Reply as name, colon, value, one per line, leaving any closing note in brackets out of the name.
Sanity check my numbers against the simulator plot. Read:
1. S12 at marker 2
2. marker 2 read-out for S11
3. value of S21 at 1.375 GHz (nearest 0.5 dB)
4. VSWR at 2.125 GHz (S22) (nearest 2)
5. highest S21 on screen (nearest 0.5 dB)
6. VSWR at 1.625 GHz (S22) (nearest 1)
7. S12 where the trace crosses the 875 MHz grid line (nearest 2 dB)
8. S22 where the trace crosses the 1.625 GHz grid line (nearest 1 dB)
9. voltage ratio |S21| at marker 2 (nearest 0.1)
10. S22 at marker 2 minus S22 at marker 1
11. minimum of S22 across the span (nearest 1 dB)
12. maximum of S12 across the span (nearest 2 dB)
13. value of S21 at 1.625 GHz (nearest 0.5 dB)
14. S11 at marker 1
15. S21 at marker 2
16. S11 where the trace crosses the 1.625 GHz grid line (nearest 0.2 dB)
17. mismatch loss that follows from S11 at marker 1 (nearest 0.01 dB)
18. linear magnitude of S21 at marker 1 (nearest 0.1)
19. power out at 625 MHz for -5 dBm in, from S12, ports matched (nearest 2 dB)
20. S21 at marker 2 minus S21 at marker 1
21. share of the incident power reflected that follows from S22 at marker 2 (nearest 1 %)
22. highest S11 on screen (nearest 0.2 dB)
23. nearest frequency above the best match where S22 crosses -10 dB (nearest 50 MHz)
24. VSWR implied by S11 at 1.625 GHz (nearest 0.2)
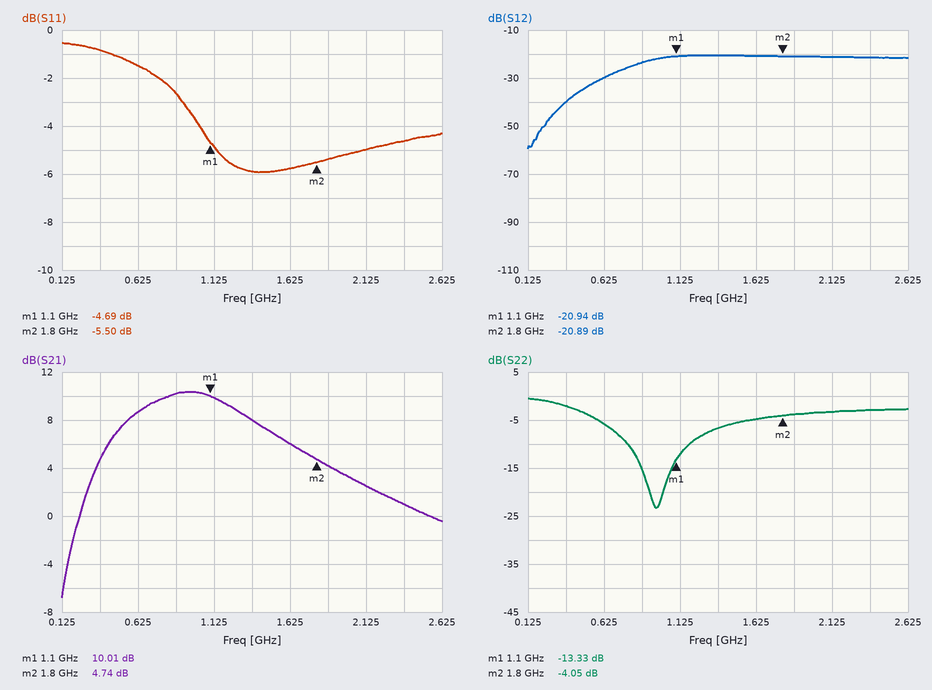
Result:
S12 at marker 2: -20.89 dB
marker 2 read-out for S11: -5.50 dB
value of S21 at 1.375 GHz: 8.0 dB
VSWR at 2.125 GHz (S22): 6
highest S21 on screen: 10.5 dB
VSWR at 1.625 GHz (S22): 4
S12 where the trace crosses the 875 MHz grid line: -24 dB
S22 where the trace crosses the 1.625 GHz grid line: -5 dB
voltage ratio |S21| at marker 2: 1.7
S22 at marker 2 minus S22 at marker 1: 9.28 dB
minimum of S22 across the span: -23 dB
maximum of S12 across the span: -20 dB
value of S21 at 1.625 GHz: 6.0 dB
S11 at marker 1: -4.69 dB
S21 at marker 2: 4.74 dB
S11 where the trace crosses the 1.625 GHz grid line: -5.8 dB
mismatch loss that follows from S11 at marker 1: 1.80 dB
linear magnitude of S21 at marker 1: 3.2
power out at 625 MHz for -5 dBm in, from S12, ports matched: -34 dBm
S21 at marker 2 minus S21 at marker 1: -5.27 dB
share of the incident power reflected that follows from S22 at marker 2: 39 %
highest S11 on screen: -0.6 dB
nearest frequency above the best match where S22 crosses -10 dB: 1.20 GHz
VSWR implied by S11 at 1.625 GHz: 3.2
